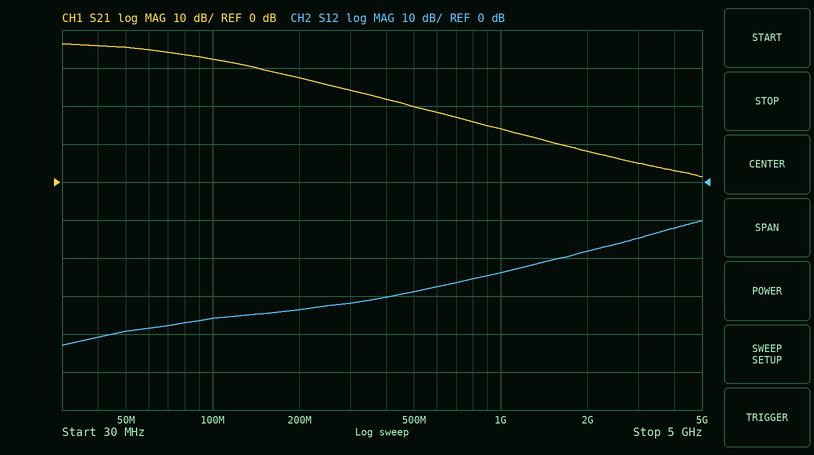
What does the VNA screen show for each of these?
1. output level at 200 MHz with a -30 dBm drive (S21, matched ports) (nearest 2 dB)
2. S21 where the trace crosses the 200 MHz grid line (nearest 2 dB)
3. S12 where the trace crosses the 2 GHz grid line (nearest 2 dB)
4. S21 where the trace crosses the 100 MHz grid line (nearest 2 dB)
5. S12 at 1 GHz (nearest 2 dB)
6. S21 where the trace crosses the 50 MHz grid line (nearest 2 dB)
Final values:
-2 dBm
28 dB
-18 dB
32 dB
-24 dB
36 dB
